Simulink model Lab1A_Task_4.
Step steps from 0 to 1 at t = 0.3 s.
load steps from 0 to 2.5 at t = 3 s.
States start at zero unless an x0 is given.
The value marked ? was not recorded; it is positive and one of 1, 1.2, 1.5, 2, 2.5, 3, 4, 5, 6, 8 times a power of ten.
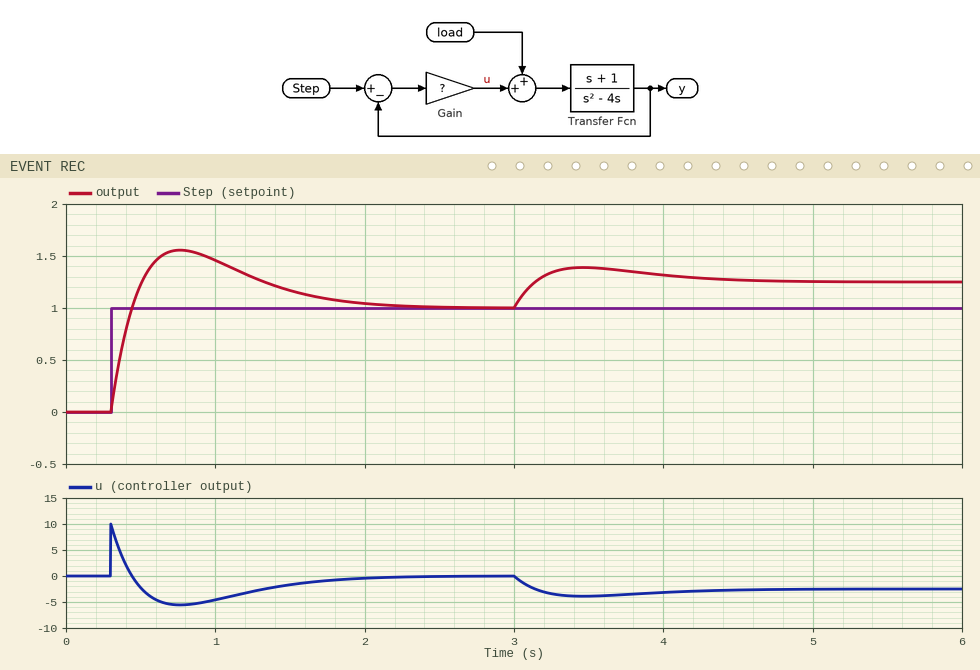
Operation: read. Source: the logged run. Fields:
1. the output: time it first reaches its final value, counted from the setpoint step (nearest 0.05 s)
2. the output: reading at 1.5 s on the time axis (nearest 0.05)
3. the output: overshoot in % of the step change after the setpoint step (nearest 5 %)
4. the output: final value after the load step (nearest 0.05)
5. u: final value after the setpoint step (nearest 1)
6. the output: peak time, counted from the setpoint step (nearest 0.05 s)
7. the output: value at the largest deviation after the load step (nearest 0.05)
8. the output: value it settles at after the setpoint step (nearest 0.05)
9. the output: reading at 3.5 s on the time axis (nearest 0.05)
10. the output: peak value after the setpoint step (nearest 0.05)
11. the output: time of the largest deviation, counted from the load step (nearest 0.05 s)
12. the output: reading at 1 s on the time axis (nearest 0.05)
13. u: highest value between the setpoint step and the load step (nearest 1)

0.15 s
1.15
55 %
1.25
0
0.45 s
1.40
1.00
1.40
1.55
0.45 s
1.45
10
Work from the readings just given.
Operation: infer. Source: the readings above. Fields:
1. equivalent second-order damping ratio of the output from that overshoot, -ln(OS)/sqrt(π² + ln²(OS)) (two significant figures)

0.19
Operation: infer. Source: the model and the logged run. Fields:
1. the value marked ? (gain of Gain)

10
